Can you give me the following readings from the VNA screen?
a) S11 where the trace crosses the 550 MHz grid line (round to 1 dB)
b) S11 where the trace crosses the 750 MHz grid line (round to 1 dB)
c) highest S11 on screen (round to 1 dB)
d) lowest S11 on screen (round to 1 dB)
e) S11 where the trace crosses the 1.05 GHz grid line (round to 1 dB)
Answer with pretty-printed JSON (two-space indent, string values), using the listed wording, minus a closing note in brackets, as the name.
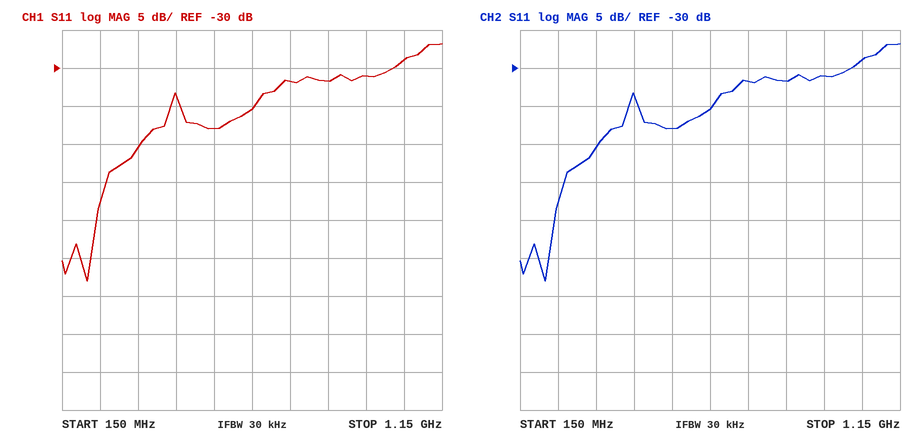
{
  "S11 where the trace crosses the 550 MHz grid line": "-38 dB",
  "S11 where the trace crosses the 750 MHz grid line": "-32 dB",
  "highest S11 on screen": "-27 dB",
  "lowest S11 on screen": "-58 dB",
  "S11 where the trace crosses the 1.05 GHz grid line": "-29 dB"
}
